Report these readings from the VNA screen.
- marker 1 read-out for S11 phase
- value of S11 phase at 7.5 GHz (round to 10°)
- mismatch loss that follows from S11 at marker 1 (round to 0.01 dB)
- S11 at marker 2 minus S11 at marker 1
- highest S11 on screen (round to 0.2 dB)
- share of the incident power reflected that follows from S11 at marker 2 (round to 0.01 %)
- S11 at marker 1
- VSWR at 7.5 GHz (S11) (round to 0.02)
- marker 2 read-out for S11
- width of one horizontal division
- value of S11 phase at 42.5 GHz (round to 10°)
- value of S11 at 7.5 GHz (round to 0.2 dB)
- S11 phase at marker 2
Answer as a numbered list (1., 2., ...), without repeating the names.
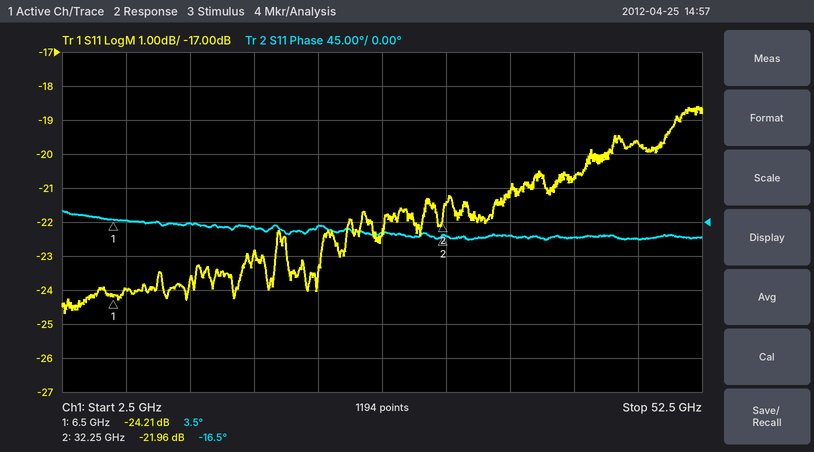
1. 3.5°
2. 0°
3. 0.02 dB
4. 2.25 dB
5. -18.6 dB
6. 0.64 %
7. -24.21 dB
8. 1.14
9. -21.96 dB
10. 5 GHz
11. -20°
12. -24.0 dB
13. -16.5°
